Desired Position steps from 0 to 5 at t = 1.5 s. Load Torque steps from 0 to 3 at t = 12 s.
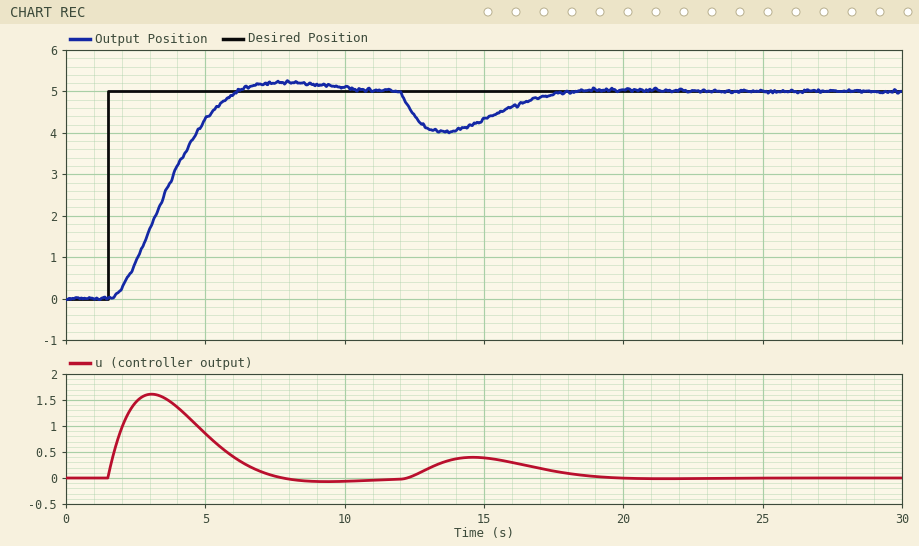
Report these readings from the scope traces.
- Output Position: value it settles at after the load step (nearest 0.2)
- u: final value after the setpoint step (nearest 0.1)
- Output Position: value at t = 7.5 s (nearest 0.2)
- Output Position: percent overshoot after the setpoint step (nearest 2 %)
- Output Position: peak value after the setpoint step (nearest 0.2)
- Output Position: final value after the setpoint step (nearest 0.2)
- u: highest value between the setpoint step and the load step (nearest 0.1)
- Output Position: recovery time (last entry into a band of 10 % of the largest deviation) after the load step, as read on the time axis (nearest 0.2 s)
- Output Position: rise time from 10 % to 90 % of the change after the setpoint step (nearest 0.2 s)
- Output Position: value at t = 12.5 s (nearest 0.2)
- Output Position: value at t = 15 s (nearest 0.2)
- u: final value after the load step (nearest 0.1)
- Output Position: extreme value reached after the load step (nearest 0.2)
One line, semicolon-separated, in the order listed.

5.0; 0.0; 5.2; 4 %; 5.2; 5.0; 1.6; 17.4 s; 3.0 s; 4.4; 4.4; 0.0; 4.0
